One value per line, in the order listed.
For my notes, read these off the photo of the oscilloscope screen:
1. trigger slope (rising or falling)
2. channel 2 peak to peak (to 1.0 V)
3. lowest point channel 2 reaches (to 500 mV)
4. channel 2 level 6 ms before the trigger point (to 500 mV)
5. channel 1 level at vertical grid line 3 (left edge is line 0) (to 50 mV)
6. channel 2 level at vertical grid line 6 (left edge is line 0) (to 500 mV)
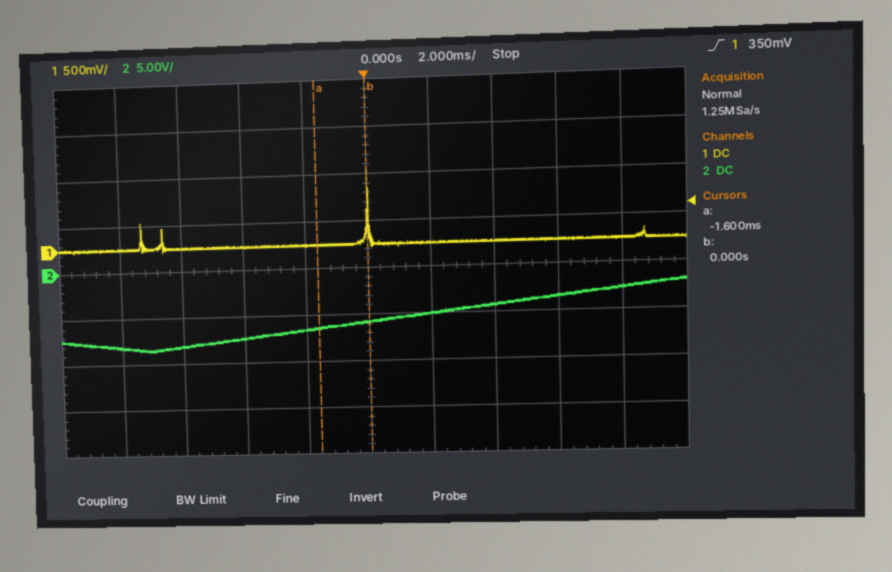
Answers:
rising
7.0 V
-8.5 V
-8.0 V
0 mV
-5.0 V
